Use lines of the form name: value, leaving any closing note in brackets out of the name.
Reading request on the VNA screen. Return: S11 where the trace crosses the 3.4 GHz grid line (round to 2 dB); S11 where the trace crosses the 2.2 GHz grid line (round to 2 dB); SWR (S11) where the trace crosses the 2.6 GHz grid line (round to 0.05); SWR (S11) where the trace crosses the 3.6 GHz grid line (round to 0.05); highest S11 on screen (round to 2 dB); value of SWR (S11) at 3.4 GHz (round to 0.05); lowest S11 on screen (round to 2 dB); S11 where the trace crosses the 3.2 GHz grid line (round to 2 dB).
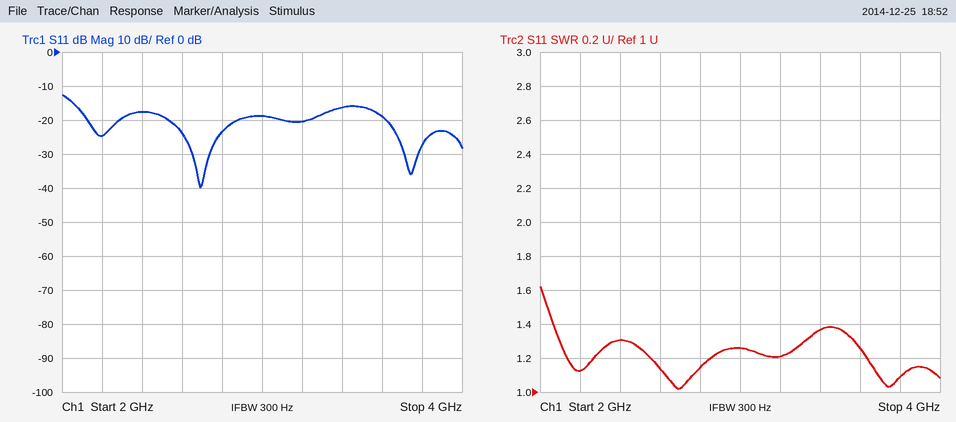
S11 where the trace crosses the 3.4 GHz grid line: -16 dB
S11 where the trace crosses the 2.2 GHz grid line: -24 dB
SWR (S11) where the trace crosses the 2.6 GHz grid line: 1.15
SWR (S11) where the trace crosses the 3.6 GHz grid line: 1.25
highest S11 on screen: -12 dB
value of SWR (S11) at 3.4 GHz: 1.35
lowest S11 on screen: -40 dB
S11 where the trace crosses the 3.2 GHz grid line: -20 dB
